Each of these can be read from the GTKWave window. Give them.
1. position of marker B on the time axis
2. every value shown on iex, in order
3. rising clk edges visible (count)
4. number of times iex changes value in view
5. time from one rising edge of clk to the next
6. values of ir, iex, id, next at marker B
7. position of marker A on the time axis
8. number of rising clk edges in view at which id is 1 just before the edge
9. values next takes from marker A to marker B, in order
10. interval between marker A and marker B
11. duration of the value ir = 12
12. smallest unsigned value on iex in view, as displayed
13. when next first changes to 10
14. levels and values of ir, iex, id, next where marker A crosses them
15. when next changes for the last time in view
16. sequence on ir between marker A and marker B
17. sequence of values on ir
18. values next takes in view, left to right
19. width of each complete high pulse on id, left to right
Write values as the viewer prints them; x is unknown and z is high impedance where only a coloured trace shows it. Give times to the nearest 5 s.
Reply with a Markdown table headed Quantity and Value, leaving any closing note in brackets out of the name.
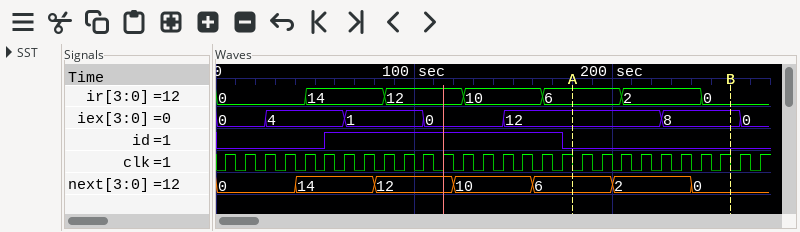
| Quantity | Value |
|---|---|
| position of marker B on the time axis | 260 s |
| every value shown on iex, in order | 0, 4, 1, 0, 12, 8, 0 |
| rising clk edges visible | 28 |
| number of times iex changes value in view | 6 |
| time from one rising edge of clk to the next | 10 s |
| values of ir, iex, id, next at marker B | ir=0, iex=8, id=0, next=0 |
| position of marker A on the time axis | 180 s |
| number of rising clk edges in view at which id is 1 just before the edge | 12 |
| values next takes from marker A to marker B, in order | 6, 2, 0 |
| interval between marker A and marker B | 80 s |
| duration of the value ir = 12 | 40 s |
| smallest unsigned value on iex in view, as displayed | 0 |
| when next first changes to 10 | 120 s |
| levels and values of ir, iex, id, next where marker A crosses them | ir=6, iex=12, id=0, next=6 |
| when next changes for the last time in view | 240 s |
| sequence on ir between marker A and marker B | 6, 2, 0 |
| sequence of values on ir | 0, 14, 12, 10, 6, 2, 0 |
| values next takes in view, left to right | 0, 14, 12, 10, 6, 2, 0 |
| width of each complete high pulse on id, left to right | 120 s |
